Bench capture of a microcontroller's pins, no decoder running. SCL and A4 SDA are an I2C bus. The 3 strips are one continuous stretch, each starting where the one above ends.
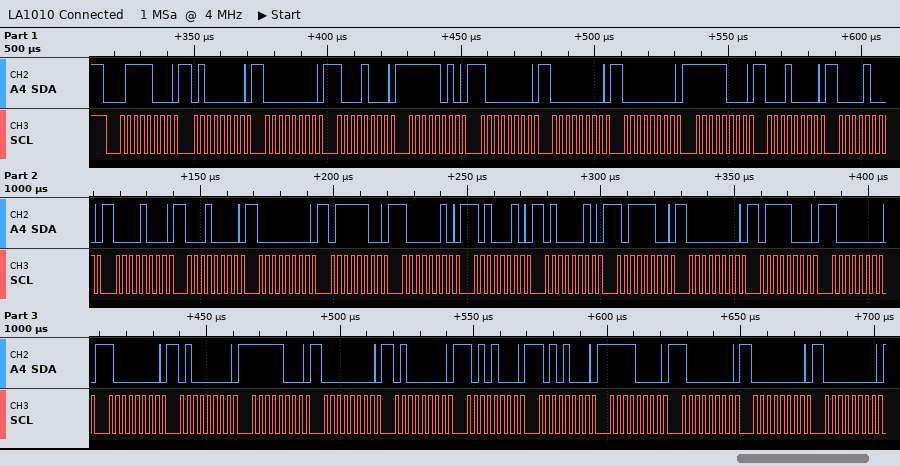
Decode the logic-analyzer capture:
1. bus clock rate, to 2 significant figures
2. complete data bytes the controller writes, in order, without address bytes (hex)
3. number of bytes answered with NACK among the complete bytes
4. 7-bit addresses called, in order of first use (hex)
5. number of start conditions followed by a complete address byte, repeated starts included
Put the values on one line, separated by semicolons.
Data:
400 kHz; 40 00 88 FA 80 00 00 F8 10 08 08 10 00 7C 82 A2 42 BC 00 78 80 80 40 F8 00 40 A8 A8 F0 80 00 00; 0; 0x3C; 1
